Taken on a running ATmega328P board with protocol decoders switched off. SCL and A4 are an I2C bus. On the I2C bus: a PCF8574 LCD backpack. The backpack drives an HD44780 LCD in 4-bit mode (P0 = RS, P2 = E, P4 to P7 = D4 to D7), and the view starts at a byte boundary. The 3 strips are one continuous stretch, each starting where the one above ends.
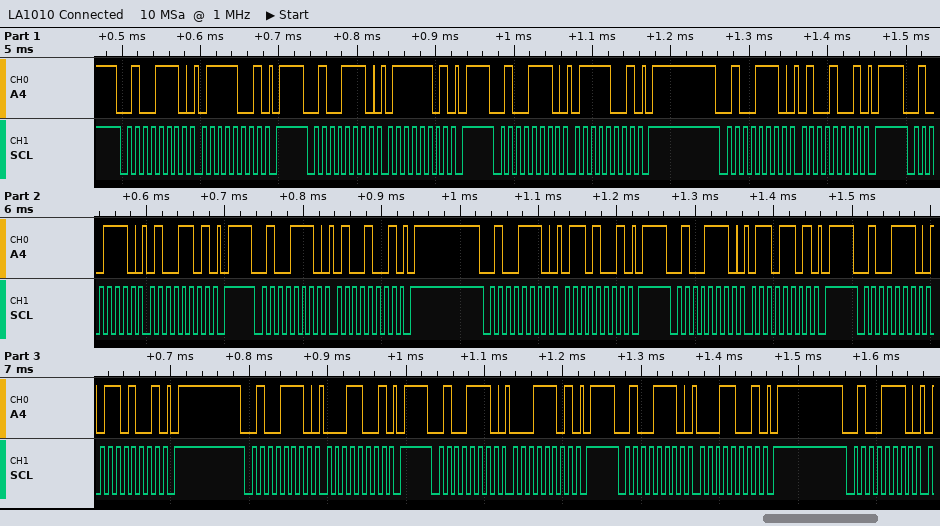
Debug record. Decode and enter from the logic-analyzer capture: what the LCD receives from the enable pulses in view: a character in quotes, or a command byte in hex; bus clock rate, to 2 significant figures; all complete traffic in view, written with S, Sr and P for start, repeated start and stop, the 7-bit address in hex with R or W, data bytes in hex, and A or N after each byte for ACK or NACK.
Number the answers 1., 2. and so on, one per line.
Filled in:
1. 't' 'a'
2. 100 kHz
3. S 27W A 79 A P S 27W A 7D A P S 27W A 79 A P S 27W A 49 A P S 27W A 4D A P S 27W A 49 A P S 27W A 69 A P S 27W A 6D A P S 27W A 69 A P S 27W A 19 A P S 27W A 1D A P S 27W A 19 A P S 27W A
